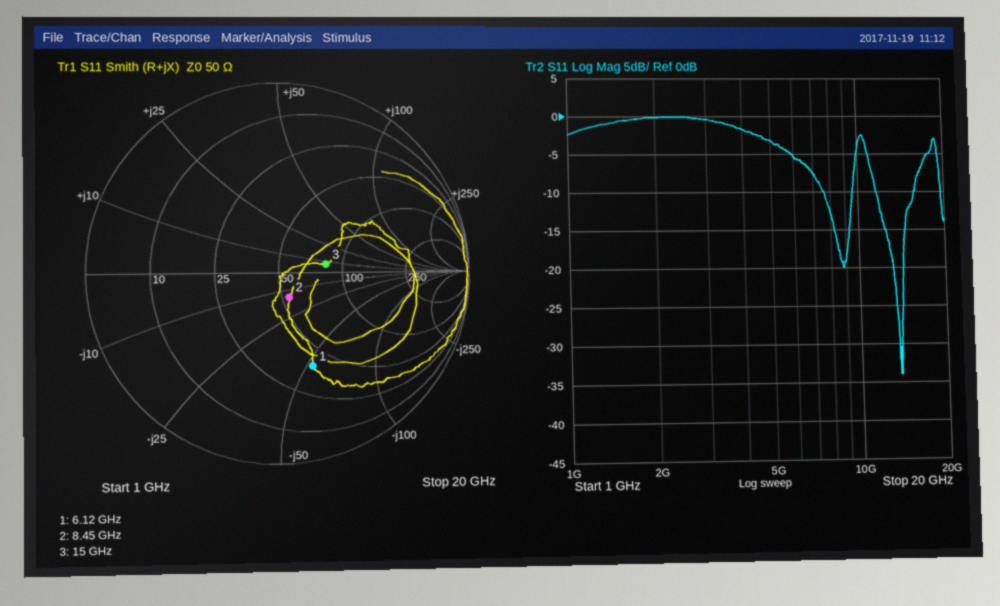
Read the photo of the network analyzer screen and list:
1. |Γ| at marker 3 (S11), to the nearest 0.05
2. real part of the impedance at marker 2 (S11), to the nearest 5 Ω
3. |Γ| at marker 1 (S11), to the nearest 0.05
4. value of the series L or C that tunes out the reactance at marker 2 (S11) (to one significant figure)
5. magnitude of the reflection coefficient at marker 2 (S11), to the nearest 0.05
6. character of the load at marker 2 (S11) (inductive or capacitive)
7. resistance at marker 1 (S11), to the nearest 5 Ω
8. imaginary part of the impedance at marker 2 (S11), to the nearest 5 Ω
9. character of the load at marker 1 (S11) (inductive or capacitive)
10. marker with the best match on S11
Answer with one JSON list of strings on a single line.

["0.25", "55 Ω", "0.50", "300 pH", "0.15", "capacitive", "40 Ω", "-15 Ω", "capacitive", "marker 2"]
